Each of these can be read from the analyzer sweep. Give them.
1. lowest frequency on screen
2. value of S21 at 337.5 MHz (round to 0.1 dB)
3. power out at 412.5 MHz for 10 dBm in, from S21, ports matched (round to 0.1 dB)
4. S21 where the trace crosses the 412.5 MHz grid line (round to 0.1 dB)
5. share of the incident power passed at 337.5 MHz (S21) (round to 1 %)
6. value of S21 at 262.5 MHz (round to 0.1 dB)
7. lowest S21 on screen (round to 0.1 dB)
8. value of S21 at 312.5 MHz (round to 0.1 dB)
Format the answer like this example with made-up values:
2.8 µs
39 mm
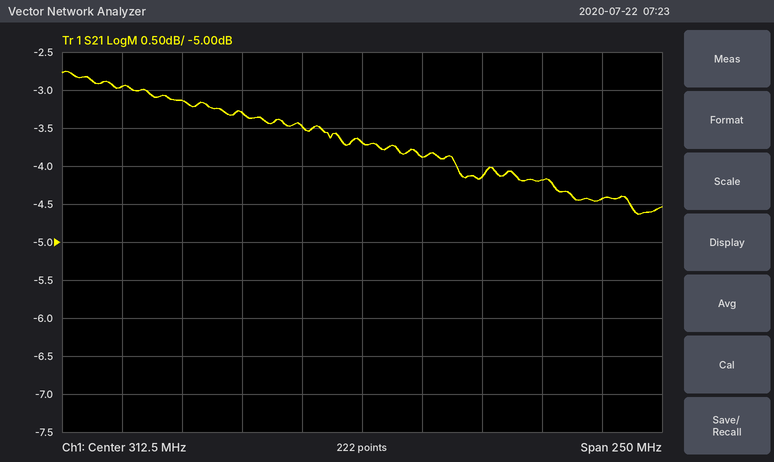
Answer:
187.5 MHz
-3.9 dB
5.6 dBm
-4.4 dB
41 %
-3.3 dB
-4.6 dB
-3.7 dB
